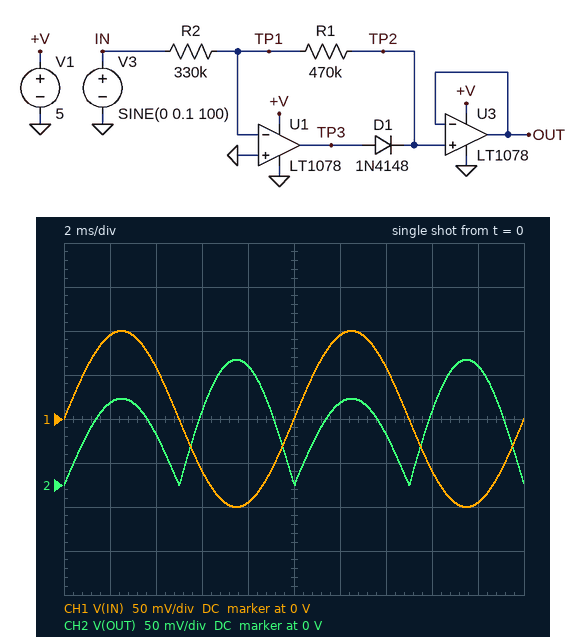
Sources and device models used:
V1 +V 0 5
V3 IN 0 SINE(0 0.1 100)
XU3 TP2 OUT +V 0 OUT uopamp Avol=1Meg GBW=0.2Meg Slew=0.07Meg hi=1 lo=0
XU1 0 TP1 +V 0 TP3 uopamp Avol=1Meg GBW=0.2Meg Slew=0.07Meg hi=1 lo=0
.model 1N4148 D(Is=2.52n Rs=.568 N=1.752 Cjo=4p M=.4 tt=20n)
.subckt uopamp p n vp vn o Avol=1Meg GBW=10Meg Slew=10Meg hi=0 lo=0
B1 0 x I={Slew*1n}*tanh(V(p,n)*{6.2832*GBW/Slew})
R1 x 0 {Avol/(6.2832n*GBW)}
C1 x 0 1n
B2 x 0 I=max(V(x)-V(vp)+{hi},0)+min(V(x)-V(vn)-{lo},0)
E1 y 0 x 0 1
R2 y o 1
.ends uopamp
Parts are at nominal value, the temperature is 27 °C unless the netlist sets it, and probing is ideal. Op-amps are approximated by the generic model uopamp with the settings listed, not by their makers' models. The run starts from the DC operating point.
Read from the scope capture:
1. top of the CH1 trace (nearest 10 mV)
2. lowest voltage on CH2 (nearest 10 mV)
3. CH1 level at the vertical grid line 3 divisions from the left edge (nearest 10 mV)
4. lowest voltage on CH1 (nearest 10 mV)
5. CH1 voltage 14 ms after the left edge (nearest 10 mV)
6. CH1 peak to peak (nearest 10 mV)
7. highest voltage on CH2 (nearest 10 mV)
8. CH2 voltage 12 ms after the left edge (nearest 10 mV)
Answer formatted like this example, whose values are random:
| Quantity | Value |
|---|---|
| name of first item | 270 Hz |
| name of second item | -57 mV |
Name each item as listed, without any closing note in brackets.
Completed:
| Quantity | Value |
|---|---|
| top of the CH1 trace | 100 mV |
| lowest voltage on CH2 | 0 V |
| CH1 level at the vertical grid line 3 divisions from the left edge | -60 mV |
| lowest voltage on CH1 | -100 mV |
| CH1 voltage 14 ms after the left edge | 60 mV |
| CH1 peak to peak | 200 mV |
| highest voltage on CH2 | 140 mV |
| CH2 voltage 12 ms after the left edge | 90 mV |
